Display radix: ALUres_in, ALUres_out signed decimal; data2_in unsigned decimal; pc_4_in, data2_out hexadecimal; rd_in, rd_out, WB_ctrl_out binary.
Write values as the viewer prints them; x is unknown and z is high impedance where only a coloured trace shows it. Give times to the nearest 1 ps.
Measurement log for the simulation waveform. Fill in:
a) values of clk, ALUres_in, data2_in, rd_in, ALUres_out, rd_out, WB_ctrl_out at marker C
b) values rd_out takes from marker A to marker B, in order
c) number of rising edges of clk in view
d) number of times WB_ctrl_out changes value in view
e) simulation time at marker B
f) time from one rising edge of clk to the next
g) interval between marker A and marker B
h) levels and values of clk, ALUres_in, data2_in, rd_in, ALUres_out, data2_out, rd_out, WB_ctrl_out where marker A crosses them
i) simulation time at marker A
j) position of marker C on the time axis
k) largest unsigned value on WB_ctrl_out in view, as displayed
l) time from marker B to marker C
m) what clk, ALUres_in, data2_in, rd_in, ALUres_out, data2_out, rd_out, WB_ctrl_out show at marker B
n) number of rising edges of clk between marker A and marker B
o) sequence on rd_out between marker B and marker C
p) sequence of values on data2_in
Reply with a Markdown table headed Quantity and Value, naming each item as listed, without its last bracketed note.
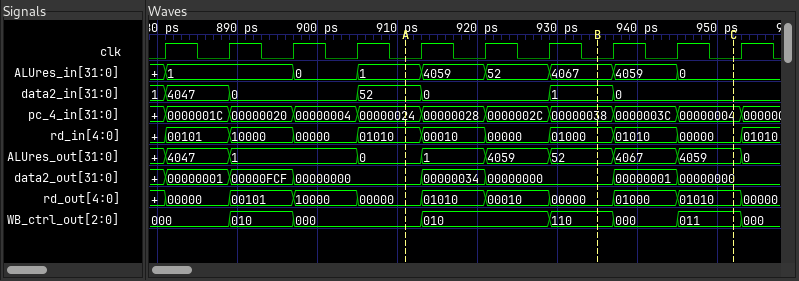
| Quantity | Value |
|---|---|
| values of clk, ALUres_in, data2_in, rd_in, ALUres_out, rd_out, WB_ctrl_out at marker C | clk=0, ALUres_in=0, data2_in=0, rd_in=00000, ALUres_out=4059, rd_out=01010, WB_ctrl_out=011 |
| values rd_out takes from marker A to marker B, in order | 00000, 01010, 00010, 00000 |
| number of rising edges of clk in view | 10 |
| number of times WB_ctrl_out changes value in view | 7 |
| simulation time at marker B | 935 ps |
| time from one rising edge of clk to the next | 8 ps |
| interval between marker A and marker B | 24 ps |
| levels and values of clk, ALUres_in, data2_in, rd_in, ALUres_out, data2_out, rd_out, WB_ctrl_out where marker A crosses them | clk=0, ALUres_in=1, data2_in=52, rd_in=01010, ALUres_out=0, data2_out=00000000, rd_out=00000, WB_ctrl_out=000 |
| simulation time at marker A | 911 ps |
| position of marker C on the time axis | 952 ps |
| largest unsigned value on WB_ctrl_out in view, as displayed | 110 |
| time from marker B to marker C | 17 ps |
| what clk, ALUres_in, data2_in, rd_in, ALUres_out, data2_out, rd_out, WB_ctrl_out show at marker B | clk=0, ALUres_in=4067, data2_in=1, rd_in=01000, ALUres_out=52, data2_out=00000000, rd_out=00000, WB_ctrl_out=110 |
| number of rising edges of clk between marker A and marker B | 3 |
| sequence on rd_out between marker B and marker C | 00000, 01000, 01010 |
| sequence of values on data2_in | 1, 4047, 0, 52, 0, 1, 0 |
